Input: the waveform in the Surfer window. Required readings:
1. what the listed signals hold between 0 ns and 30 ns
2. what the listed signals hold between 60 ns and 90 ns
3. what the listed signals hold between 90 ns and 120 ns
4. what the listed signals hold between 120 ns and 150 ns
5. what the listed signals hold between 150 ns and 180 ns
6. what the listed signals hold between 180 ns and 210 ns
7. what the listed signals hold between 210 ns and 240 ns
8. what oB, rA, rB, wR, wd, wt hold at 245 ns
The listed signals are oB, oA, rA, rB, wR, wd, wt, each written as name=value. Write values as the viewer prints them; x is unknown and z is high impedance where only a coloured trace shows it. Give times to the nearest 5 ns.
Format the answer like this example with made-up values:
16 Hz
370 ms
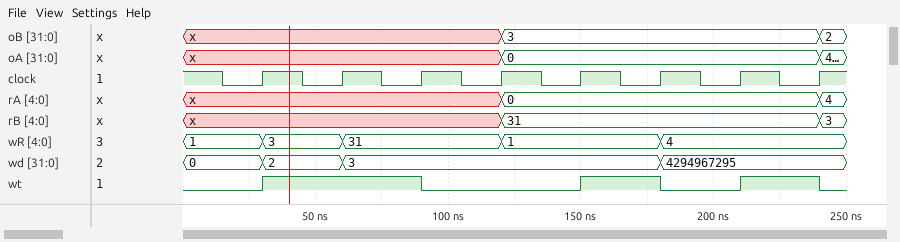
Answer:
oB=x, oA=x, rA=x, rB=x, wR=1, wd=0, wt=0
oB=x, oA=x, rA=x, rB=x, wR=31, wd=3, wt=1
oB=x, oA=x, rA=x, rB=x, wR=31, wd=3, wt=0
oB=3, oA=0, rA=0, rB=31, wR=1, wd=3, wt=0
oB=3, oA=0, rA=0, rB=31, wR=1, wd=3, wt=1
oB=3, oA=0, rA=0, rB=31, wR=4, wd=4294967295, wt=0
oB=3, oA=0, rA=0, rB=31, wR=4, wd=4294967295, wt=1
oB=2, rA=4, rB=3, wR=4, wd=4294967295, wt=0
